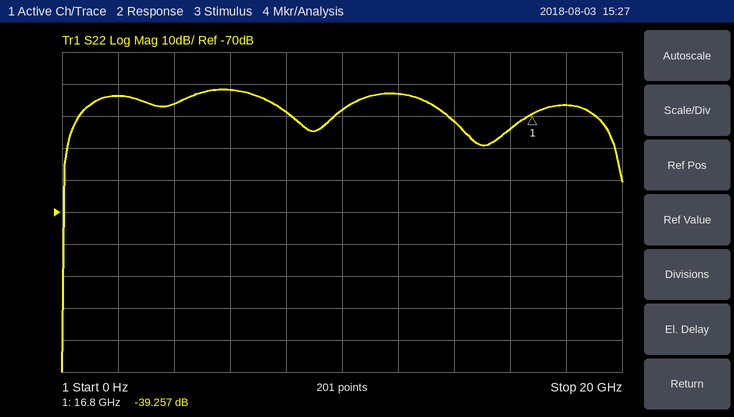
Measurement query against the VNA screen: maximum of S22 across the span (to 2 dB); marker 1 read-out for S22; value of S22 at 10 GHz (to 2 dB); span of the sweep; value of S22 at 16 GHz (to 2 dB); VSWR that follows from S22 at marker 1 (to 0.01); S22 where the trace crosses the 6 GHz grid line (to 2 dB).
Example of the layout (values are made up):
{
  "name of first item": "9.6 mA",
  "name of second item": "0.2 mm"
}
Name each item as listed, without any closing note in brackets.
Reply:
{
  "maximum of S22 across the span": "-32 dB",
  "marker 1 read-out for S22": "-39.257 dB",
  "value of S22 at 10 GHz": "-38 dB",
  "span of the sweep": "20 GHz",
  "value of S22 at 16 GHz": "-44 dB",
  "VSWR that follows from S22 at marker 1": "1.02",
  "S22 where the trace crosses the 6 GHz grid line": "-32 dB"
}
